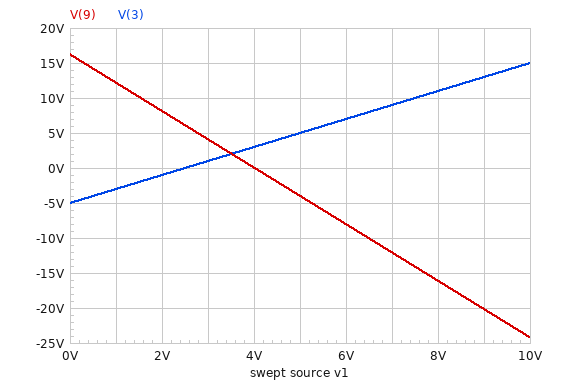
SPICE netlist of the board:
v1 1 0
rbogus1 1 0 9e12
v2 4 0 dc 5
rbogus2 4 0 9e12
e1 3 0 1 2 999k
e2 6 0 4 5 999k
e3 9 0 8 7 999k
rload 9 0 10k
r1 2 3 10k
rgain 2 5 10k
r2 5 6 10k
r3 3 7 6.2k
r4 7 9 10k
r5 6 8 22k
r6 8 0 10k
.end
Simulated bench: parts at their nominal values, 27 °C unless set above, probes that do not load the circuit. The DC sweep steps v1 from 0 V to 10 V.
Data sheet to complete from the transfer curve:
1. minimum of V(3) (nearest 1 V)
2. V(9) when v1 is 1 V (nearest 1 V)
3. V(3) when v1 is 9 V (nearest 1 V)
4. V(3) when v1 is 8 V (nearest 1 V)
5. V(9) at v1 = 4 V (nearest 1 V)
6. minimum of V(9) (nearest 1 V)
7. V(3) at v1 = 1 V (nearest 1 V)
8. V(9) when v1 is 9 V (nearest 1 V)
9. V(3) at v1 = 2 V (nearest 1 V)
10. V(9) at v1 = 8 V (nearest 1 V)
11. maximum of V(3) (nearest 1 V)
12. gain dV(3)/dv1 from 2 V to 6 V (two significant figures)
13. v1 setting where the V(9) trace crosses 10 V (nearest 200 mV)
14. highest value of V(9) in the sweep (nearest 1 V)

-5 V
12 V
13 V
11 V
0 V
-24 V
-3 V
-20 V
-1 V
-16 V
15 V
2.0 V/V
1.6 V
16 V
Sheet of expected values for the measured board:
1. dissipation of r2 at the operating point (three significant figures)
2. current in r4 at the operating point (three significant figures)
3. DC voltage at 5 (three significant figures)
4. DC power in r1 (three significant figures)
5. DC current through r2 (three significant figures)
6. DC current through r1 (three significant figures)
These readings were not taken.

2.50 mW
1.31 mA
5.00 V
2.50 mW
500 µA
500 µA
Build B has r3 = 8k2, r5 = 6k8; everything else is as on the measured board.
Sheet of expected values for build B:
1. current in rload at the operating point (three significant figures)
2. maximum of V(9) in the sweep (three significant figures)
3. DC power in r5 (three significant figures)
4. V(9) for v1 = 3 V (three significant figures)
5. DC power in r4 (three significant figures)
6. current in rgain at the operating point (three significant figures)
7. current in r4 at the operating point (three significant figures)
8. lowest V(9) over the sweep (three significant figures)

1.93 mA
19.3 V
2.41 mW
8.03 V
17.8 mW
500 µA
1.34 mA
-18.3 V
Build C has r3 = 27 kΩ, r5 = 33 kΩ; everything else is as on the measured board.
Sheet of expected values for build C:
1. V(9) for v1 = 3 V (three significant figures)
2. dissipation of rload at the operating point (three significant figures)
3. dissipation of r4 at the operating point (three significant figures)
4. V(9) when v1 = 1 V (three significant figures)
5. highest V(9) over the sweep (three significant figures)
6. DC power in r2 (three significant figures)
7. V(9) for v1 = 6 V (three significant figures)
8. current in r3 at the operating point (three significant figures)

1.86 V
2.54 mW
736 µW
3.98 V
5.04 V
2.50 mW
-1.32 V
271 µA
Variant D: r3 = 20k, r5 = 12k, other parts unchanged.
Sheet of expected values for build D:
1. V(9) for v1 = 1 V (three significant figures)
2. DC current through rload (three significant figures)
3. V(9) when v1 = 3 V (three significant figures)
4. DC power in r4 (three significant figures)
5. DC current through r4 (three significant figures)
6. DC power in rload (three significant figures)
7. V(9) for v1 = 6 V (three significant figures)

7.64 V
932 µA
4.27 V
2.28 mW
477 µA
8.68 mW
-773 mV
